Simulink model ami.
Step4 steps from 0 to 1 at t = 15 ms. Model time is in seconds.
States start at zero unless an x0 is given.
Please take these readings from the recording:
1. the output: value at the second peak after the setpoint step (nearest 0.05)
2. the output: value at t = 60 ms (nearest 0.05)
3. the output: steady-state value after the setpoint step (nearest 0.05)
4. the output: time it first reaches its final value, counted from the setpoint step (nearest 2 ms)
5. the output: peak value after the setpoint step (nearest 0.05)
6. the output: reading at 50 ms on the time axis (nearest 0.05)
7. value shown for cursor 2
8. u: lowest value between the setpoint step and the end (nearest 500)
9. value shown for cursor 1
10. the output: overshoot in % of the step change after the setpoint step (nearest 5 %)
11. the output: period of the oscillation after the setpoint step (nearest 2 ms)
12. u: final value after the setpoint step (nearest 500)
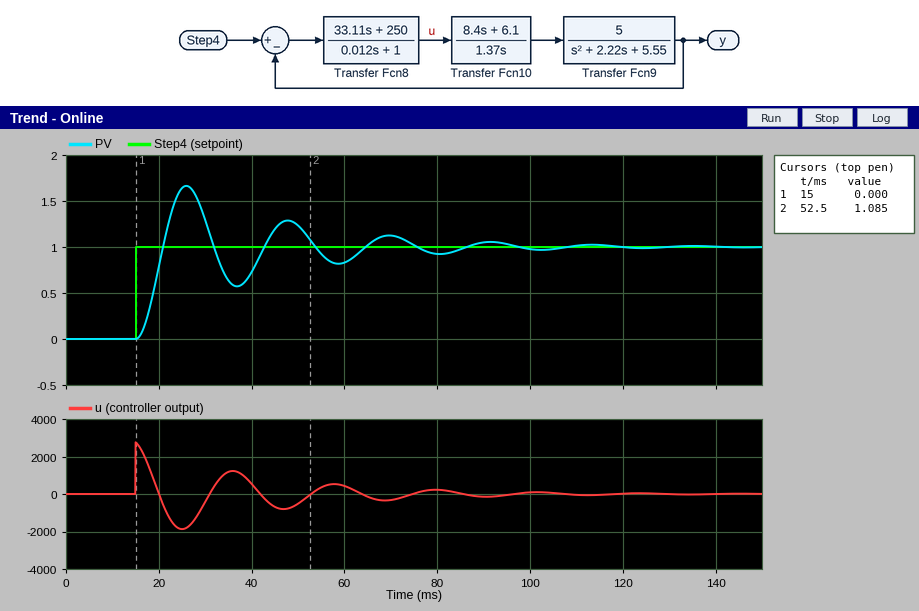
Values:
1.30
0.85
1.00
6 ms
1.65
1.25
1.085
-2000
0.000
65 %
22 ms
0
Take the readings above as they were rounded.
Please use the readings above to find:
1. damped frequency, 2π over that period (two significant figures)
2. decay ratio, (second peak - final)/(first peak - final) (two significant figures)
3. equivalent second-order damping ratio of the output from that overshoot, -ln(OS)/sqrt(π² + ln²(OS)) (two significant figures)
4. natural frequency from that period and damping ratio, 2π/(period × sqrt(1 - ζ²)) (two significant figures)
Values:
0.29 rad/ms
0.46
0.14
0.29 rad/ms
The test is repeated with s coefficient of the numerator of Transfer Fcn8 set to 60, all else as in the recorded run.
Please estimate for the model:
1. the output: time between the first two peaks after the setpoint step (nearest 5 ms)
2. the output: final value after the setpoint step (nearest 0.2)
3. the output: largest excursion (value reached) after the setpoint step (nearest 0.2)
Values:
15 ms
1.0
1.8
